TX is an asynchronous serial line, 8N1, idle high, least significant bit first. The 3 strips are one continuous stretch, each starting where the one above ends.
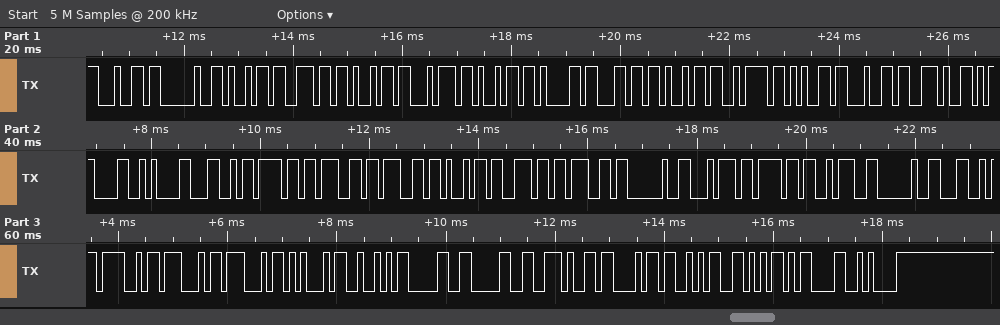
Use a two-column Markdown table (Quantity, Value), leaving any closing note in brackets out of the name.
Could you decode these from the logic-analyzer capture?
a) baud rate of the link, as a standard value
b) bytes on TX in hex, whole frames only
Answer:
| Quantity | Value |
|---|---|
| baud rate of the link, as a standard value | 9600 baud |
| bytes on TX in hex, whole frames only | 64 20 69 6E 69 74 69 61 6C 69 7A 65 64 2E 0D 0A 4C 6F 67 67 69 6E 67 20 74 6F 3A 20 4C 4F 47 47 45 52 30 30 2E 43 53 56 0D 0A |
